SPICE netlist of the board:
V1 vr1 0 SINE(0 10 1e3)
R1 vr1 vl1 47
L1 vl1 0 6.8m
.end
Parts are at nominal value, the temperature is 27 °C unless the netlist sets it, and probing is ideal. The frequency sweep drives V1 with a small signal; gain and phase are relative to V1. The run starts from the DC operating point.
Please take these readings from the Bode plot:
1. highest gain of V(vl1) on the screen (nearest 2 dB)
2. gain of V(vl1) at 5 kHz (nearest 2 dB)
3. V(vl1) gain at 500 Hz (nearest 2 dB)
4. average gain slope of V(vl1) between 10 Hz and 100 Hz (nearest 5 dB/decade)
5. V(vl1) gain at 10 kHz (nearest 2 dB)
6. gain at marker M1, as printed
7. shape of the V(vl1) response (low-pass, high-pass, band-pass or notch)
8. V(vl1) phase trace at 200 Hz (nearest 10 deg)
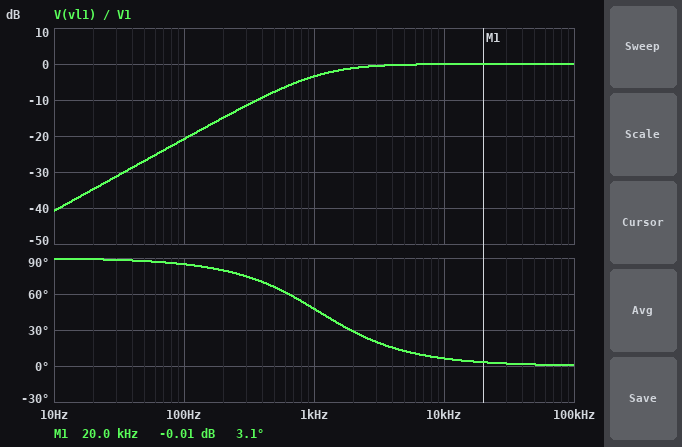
0 dB
0 dB
-8 dB
20 dB/decade
0 dB
-0.01 dB
high-pass
80 deg
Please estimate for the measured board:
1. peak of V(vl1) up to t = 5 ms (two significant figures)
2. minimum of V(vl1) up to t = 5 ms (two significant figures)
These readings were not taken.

6.7 V
-6.8 V
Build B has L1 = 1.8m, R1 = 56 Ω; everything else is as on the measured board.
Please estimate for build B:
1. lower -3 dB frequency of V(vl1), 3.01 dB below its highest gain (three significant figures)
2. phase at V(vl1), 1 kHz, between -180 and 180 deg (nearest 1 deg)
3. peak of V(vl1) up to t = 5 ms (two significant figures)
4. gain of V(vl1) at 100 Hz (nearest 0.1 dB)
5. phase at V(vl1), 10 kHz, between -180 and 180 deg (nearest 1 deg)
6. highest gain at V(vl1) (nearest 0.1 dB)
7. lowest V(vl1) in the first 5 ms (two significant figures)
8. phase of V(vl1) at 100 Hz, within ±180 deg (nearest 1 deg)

4.95 kHz
79 deg
2.0 V
-33.9 dB
26 deg
0 dB
-2.0 V
89 deg
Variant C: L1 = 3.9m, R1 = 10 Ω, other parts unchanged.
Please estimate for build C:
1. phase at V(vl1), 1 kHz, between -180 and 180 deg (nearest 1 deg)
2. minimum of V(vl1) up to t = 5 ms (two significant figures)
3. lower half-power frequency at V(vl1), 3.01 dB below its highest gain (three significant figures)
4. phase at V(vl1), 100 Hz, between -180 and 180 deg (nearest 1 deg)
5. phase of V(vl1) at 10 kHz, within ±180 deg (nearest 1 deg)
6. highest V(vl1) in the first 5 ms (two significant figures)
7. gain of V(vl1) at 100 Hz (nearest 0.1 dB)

22 deg
-9.9 V
408 Hz
76 deg
2 deg
9.3 V
-12.5 dB
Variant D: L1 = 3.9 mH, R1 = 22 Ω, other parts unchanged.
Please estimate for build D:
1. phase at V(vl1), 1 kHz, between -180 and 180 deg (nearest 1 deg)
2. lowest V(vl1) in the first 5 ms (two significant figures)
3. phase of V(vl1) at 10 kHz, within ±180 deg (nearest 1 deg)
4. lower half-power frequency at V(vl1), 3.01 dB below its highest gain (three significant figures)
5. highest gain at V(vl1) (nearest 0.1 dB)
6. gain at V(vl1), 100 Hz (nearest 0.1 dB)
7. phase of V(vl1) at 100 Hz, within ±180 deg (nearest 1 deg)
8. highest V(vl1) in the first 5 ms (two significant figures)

42 deg
-7.6 V
5 deg
898 Hz
0 dB
-19.1 dB
84 deg
7.4 V
